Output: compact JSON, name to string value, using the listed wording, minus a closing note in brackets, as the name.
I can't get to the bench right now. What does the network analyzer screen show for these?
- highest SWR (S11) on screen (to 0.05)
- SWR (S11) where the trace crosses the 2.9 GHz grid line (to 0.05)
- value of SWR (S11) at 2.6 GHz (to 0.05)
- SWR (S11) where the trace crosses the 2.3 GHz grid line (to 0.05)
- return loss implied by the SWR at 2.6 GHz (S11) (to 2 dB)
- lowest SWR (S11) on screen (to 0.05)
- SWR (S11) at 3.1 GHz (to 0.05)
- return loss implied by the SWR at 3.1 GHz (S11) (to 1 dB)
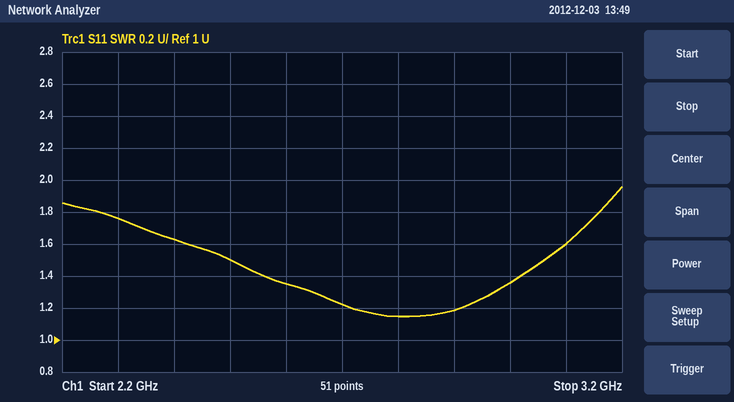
{"highest SWR (S11) on screen": "1.95", "SWR (S11) where the trace crosses the 2.9 GHz grid line": "1.20", "value of SWR (S11) at 2.6 GHz": "1.35", "SWR (S11) where the trace crosses the 2.3 GHz grid line": "1.75", "return loss implied by the SWR at 2.6 GHz (S11)": "16 dB", "lowest SWR (S11) on screen": "1.15", "SWR (S11) at 3.1 GHz": "1.60", "return loss implied by the SWR at 3.1 GHz (S11)": "13 dB"}
